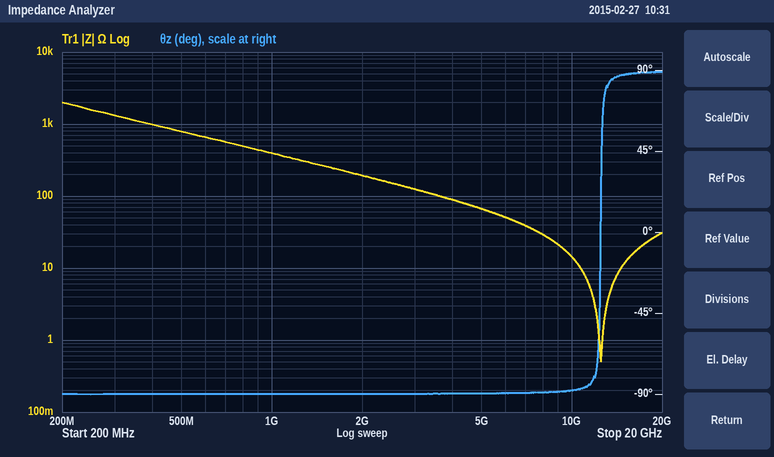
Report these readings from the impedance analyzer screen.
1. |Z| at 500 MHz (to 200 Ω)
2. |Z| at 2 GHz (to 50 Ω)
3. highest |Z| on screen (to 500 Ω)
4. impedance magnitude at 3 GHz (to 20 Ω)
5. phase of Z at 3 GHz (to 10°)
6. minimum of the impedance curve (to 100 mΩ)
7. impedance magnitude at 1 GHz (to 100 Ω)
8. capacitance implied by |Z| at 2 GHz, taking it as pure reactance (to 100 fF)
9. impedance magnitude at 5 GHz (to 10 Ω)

800 Ω
200 Ω
2.0 kΩ
120 Ω
-90°
500 mΩ
400 Ω
400 fF
70 Ω
